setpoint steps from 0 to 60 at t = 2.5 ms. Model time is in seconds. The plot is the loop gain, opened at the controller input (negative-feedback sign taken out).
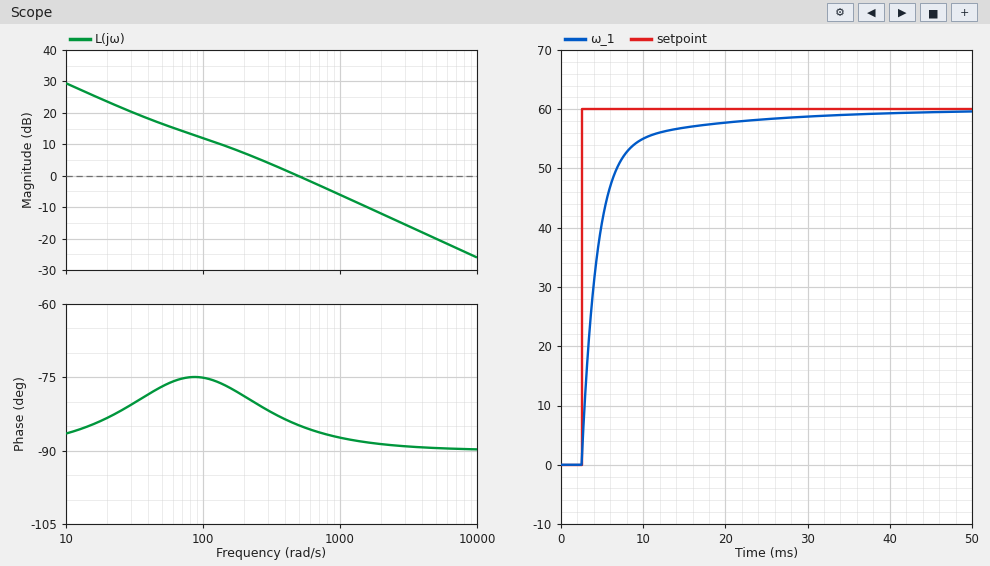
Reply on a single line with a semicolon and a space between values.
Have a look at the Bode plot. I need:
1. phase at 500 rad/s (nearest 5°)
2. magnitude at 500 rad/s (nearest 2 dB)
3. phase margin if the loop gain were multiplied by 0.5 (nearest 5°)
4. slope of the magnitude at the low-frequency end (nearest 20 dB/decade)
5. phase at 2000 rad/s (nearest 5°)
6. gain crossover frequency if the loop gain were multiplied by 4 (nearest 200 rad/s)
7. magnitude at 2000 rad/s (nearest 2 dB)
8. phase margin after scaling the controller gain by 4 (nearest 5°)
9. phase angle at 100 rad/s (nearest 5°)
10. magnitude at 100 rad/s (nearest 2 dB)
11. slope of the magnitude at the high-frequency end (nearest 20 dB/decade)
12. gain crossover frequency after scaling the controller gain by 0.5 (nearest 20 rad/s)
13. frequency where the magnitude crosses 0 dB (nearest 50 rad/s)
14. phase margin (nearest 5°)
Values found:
-85°; 0 dB; 100°; -20 dB/decade; -90°; 2000 rad/s; -12 dB; 90°; -75°; 12 dB; -20 dB/decade; 240 rad/s; 500 rad/s; 95°
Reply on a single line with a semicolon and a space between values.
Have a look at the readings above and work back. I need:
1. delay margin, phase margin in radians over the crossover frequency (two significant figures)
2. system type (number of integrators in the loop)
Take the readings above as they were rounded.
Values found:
0.0033 s; 1
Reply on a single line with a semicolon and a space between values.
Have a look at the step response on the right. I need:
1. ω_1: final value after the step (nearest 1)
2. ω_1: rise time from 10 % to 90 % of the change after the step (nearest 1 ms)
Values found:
60; 6 ms
